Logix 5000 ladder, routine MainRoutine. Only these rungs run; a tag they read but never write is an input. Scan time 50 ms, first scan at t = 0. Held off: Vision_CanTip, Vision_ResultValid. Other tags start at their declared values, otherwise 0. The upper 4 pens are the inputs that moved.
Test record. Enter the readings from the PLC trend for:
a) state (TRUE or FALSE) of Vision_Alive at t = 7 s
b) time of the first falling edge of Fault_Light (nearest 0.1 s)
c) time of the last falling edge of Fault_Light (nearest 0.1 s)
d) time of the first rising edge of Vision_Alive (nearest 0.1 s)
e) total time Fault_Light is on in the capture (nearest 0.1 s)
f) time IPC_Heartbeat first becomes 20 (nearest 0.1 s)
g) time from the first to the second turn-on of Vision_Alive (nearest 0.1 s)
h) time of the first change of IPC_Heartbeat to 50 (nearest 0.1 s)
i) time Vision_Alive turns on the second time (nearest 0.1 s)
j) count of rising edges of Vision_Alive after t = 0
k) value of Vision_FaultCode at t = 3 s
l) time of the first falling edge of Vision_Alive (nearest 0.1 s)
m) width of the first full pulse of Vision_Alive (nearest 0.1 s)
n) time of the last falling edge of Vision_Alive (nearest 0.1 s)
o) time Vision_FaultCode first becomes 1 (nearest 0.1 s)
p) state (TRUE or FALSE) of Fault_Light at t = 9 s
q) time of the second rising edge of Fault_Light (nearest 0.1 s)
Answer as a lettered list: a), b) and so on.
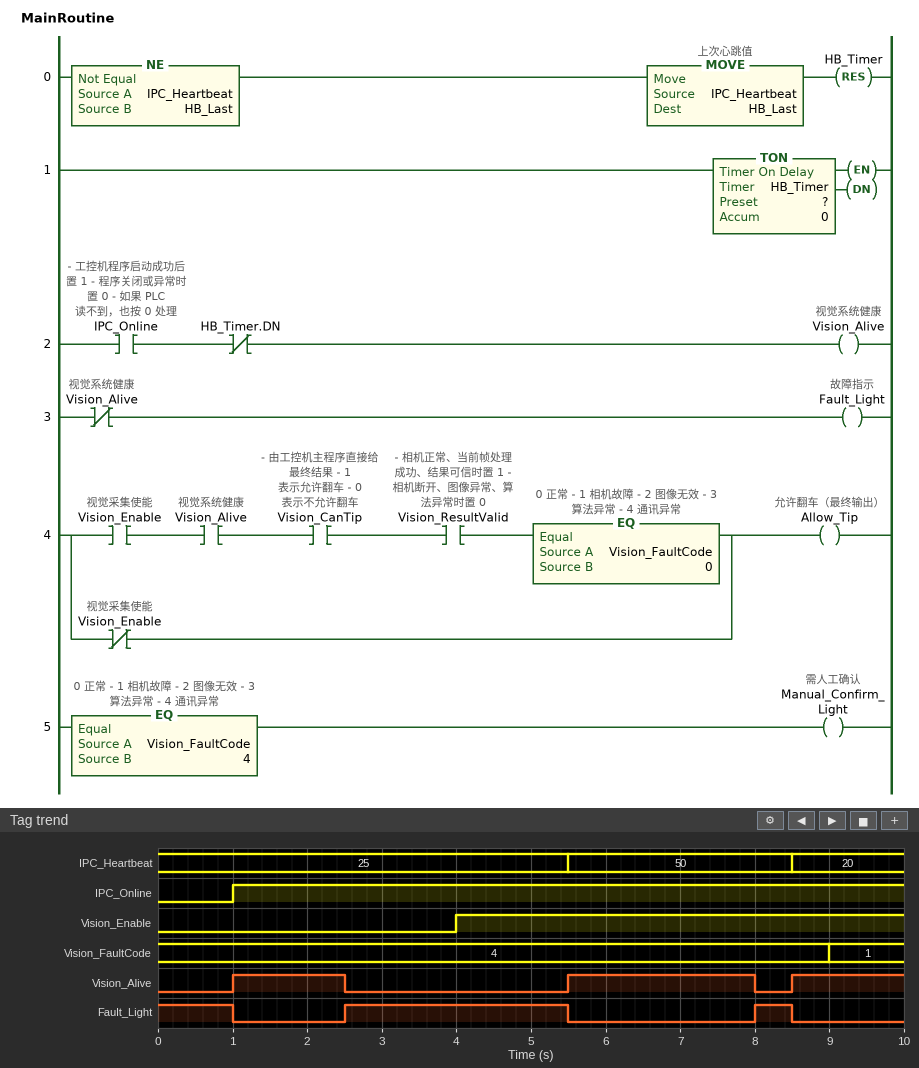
a) TRUE
b) 1.0 s
c) 8.5 s
d) 1.0 s
e) 4.5 s
f) 8.5 s
g) 4.5 s
h) 5.5 s
i) 5.5 s
j) 3
k) 4
l) 2.5 s
m) 1.5 s
n) 8.0 s
o) 9.0 s
p) FALSE
q) 8.0 s
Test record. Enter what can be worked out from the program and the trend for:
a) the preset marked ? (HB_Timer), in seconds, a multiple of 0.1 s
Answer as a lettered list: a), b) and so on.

a) 2.5 s
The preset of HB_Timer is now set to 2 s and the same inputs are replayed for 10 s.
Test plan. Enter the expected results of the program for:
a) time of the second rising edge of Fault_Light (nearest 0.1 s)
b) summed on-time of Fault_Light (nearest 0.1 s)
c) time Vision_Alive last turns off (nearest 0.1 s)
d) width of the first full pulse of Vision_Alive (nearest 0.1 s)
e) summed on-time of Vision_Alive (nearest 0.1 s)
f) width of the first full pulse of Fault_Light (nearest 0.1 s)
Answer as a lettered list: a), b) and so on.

a) 7.5 s
b) 5.5 s
c) 7.5 s
d) 1.0 s
e) 4.5 s
f) 3.5 s
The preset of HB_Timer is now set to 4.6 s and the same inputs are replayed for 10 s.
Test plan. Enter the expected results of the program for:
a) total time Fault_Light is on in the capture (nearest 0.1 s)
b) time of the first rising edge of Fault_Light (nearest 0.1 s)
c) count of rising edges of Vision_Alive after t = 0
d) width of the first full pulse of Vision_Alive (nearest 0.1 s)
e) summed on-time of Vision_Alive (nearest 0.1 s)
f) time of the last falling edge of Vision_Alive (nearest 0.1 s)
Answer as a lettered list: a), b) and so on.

a) 1.9 s
b) 4.6 s
c) 2
d) 3.6 s
e) 8.1 s
f) 4.6 s
